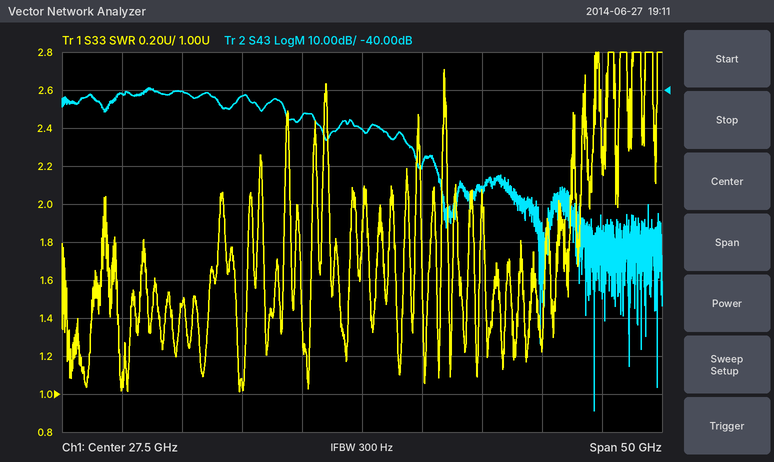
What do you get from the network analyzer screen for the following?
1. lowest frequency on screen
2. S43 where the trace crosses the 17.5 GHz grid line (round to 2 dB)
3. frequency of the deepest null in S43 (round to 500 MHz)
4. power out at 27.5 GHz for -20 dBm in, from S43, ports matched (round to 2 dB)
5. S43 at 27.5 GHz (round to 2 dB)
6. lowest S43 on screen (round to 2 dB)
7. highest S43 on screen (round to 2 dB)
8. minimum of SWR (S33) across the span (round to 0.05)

2.5 GHz
-42 dB
47.0 GHz
-70 dBm
-50 dB
-124 dB
-40 dB
1.00
